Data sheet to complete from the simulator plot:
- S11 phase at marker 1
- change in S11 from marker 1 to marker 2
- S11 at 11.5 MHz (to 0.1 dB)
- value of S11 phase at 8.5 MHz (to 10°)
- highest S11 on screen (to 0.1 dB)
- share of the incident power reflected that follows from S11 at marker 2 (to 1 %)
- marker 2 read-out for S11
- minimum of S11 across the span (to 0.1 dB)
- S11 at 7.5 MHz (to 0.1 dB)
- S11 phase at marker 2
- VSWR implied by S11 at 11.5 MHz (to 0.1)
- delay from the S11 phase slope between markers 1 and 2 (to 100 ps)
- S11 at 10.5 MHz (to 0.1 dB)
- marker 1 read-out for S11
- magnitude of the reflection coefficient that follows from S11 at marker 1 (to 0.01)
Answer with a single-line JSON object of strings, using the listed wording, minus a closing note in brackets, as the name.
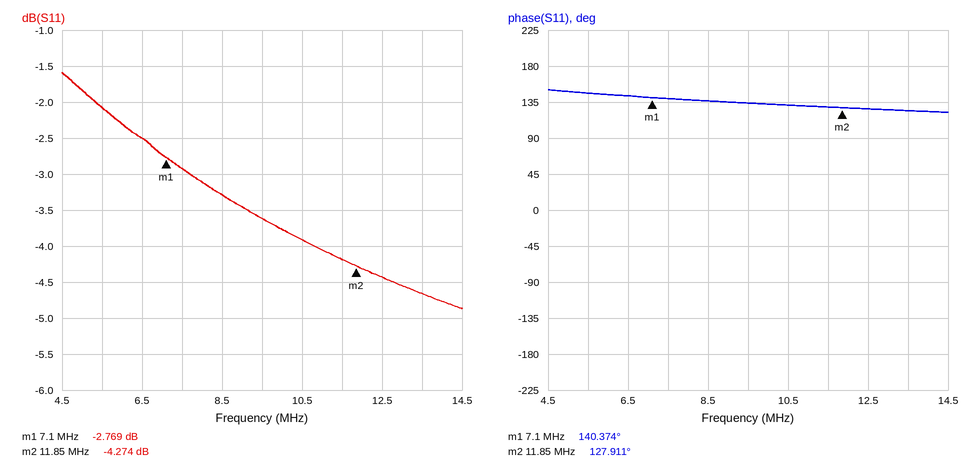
{"S11 phase at marker 1": "140.374°", "change in S11 from marker 1 to marker 2": "-1.505 dB", "S11 at 11.5 MHz": "-4.2 dB", "value of S11 phase at 8.5 MHz": "140°", "highest S11 on screen": "-1.6 dB", "share of the incident power reflected that follows from S11 at marker 2": "37 %", "marker 2 read-out for S11": "-4.274 dB", "minimum of S11 across the span": "-4.9 dB", "S11 at 7.5 MHz": "-2.9 dB", "S11 phase at marker 2": "127.911°", "VSWR implied by S11 at 11.5 MHz": "4.2", "delay from the S11 phase slope between markers 1 and 2": "7.3 ns", "S11 at 10.5 MHz": "-3.9 dB", "marker 1 read-out for S11": "-2.769 dB", "magnitude of the reflection coefficient that follows from S11 at marker 1": "0.73"}
